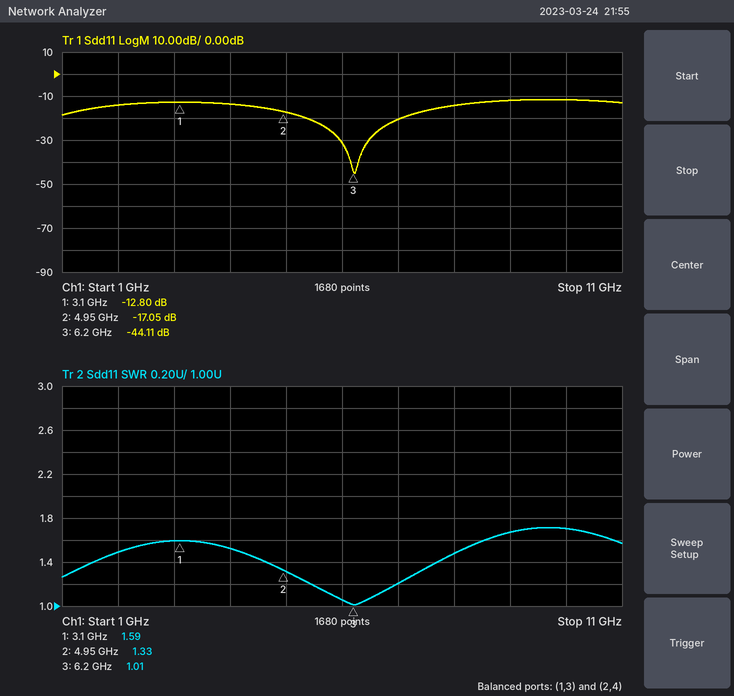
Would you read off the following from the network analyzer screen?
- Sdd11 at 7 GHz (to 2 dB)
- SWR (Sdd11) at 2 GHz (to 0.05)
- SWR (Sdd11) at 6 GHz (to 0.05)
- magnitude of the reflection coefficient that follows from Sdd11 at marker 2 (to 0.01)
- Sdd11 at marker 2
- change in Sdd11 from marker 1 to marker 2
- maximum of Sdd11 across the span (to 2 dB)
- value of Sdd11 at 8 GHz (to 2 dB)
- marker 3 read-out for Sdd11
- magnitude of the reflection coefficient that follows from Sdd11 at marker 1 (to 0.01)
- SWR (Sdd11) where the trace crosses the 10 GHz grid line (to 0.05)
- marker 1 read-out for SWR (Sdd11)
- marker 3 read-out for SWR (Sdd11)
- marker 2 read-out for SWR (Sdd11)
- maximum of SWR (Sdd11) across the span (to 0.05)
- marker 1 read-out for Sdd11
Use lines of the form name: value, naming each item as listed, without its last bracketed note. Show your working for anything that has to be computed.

Sdd11 at 7 GHz: -20 dB
SWR (Sdd11) at 2 GHz: 1.50
SWR (Sdd11) at 6 GHz: 1.05
magnitude of the reflection coefficient that follows from Sdd11 at marker 2: 10^(-17.05/20) ≈ 0.14
Sdd11 at marker 2: -17.05 dB
change in Sdd11 from marker 1 to marker 2: -17.05 − (-12.8) = -4.25 dB
maximum of Sdd11 across the span: -12 dB
value of Sdd11 at 8 GHz: -14 dB
marker 3 read-out for Sdd11: -44.11 dB
magnitude of the reflection coefficient that follows from Sdd11 at marker 1: 10^(-12.8/20) ≈ 0.23
SWR (Sdd11) where the trace crosses the 10 GHz grid line: 1.70
marker 1 read-out for SWR: 1.59
marker 3 read-out for SWR: 1.01
marker 2 read-out for SWR: 1.33
maximum of SWR (Sdd11) across the span: 1.70
marker 1 read-out for Sdd11: -12.80 dB
